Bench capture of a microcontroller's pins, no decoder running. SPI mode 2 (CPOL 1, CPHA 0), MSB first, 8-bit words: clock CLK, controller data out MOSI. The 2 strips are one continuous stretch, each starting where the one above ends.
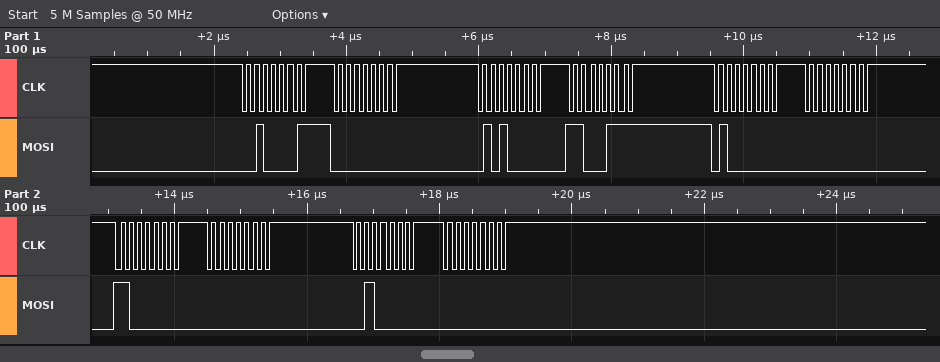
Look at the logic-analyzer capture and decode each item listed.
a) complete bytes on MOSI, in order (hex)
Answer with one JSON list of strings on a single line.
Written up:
["21 00 50 C7 40 00 C0 00 20 00"]
